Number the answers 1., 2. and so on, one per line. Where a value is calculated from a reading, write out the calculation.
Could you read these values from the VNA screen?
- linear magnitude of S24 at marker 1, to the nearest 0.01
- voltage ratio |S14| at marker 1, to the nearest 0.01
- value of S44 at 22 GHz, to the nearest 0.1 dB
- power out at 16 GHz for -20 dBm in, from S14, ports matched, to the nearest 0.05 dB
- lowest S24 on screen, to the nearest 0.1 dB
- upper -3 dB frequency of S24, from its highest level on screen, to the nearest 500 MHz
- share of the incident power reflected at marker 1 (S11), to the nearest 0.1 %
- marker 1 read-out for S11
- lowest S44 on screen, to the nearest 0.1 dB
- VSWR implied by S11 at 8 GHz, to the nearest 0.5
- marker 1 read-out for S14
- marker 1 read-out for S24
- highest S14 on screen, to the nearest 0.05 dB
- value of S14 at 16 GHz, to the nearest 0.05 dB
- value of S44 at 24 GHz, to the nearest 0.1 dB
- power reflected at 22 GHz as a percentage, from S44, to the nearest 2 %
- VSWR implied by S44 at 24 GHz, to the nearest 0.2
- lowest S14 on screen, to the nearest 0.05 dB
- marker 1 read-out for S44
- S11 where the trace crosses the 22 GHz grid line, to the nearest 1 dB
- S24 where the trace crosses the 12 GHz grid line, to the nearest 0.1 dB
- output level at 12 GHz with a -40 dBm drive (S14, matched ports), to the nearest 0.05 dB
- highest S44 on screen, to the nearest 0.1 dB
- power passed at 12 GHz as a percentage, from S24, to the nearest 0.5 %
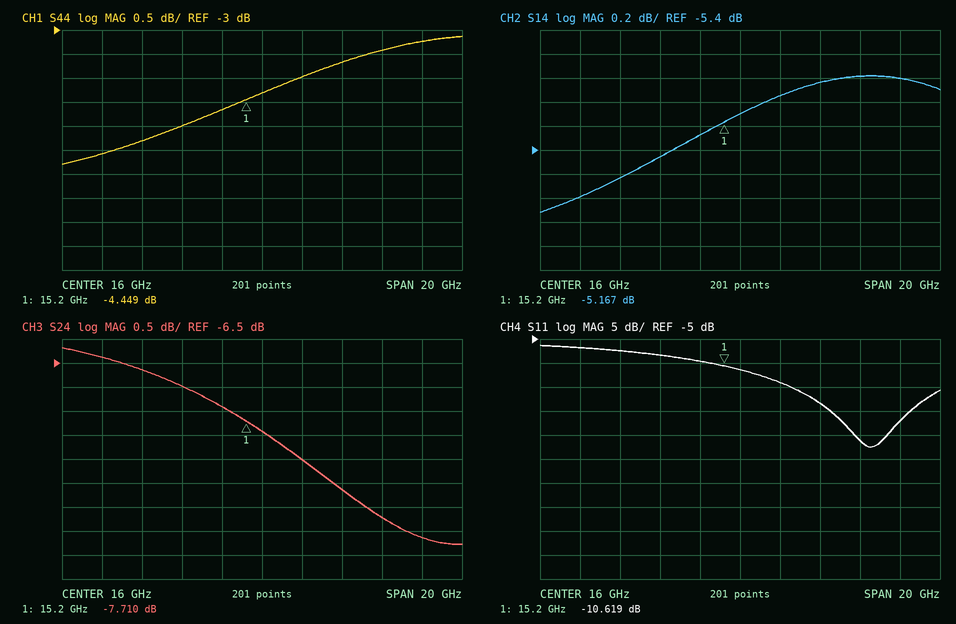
1. 10^(-7.71/20) ≈ 0.41
2. 10^(-5.167/20) ≈ 0.55
3. -3.4 dB
4. -20 dBm + (-5.10 dB) = -25.10 dBm
5. -10.3 dB
6. 20.0 GHz
7. 10^(-10.619/10) ≈ 8.7 %
8. -10.619 dB
9. -5.8 dB
10. |Γ| = 10^(-7/20) = 0.4467; VSWR = (1 + 0.4467)/(1 − 0.4467) ≈ 2.61, so 2.5 to the nearest 0.5
11. -5.167 dB
12. -7.710 dB
13. -4.80 dB
14. -5.10 dB
15. -3.2 dB
16. 10^(-3.4/10) ≈ 46 %
17. |Γ| = 10^(-3.2/20) = 0.6918; VSWR = (1 + 0.6918)/(1 − 0.6918) ≈ 5.49, so 5.4 to the nearest 0.2
18. -5.90 dB
19. -4.449 dB
20. -26 dB
21. -7.0 dB
22. -40 dBm + (-5.45 dB) = -45.45 dBm
23. -3.1 dB
24. 10^(-7/10) ≈ 20.0 %
